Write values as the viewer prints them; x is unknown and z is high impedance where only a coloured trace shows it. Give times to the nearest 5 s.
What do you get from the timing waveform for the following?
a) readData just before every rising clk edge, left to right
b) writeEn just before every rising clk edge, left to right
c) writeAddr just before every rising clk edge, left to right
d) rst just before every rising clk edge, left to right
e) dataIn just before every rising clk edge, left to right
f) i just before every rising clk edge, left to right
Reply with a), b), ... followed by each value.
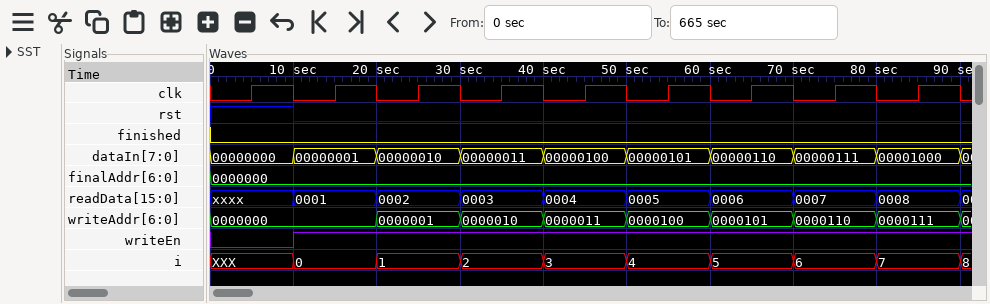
a) xxxx, 0001, 0002, 0003, 0004, 0005, 0006, 0007, 0008
b) 0 1 1 1 1 1 1 1 1
c) 0000000, 0000000, 0000001, 0000010, 0000011, 0000100, 0000101, 0000110, 0000111
d) 1 0 0 0 0 0 0 0 0
e) 00000000, 00000001, 00000010, 00000011, 00000100, 00000101, 00000110, 00000111, 00001000
f) XXX, 0, 1, 2, 3, 4, 5, 6, 7
